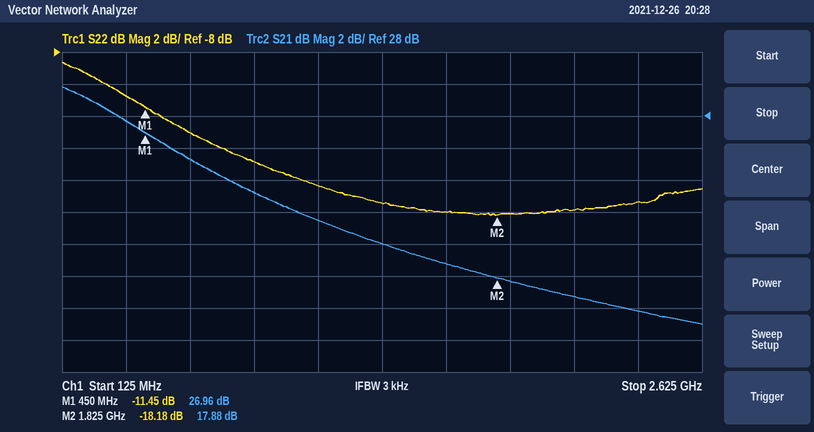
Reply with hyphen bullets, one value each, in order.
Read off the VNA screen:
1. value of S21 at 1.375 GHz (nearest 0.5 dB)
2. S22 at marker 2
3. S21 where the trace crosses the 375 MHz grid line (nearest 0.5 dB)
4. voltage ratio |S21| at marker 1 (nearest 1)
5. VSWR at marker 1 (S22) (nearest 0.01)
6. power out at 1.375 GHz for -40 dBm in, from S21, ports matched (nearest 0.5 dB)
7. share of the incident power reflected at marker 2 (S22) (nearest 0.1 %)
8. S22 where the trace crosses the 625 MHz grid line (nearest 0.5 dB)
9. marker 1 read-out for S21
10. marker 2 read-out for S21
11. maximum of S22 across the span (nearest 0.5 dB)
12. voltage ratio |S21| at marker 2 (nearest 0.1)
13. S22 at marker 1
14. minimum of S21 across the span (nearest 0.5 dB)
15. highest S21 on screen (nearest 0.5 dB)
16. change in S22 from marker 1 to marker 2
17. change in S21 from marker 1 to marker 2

- 20.0 dB
- -18.18 dB
- 27.5 dB
- 22
- 1.73
- -20.0 dBm
- 1.5 %
- -13.0 dB
- 26.96 dB
- 17.88 dB
- -8.5 dB
- 7.8
- -11.45 dB
- 15.0 dB
- 30.0 dB
- -6.73 dB
- -9.08 dB
